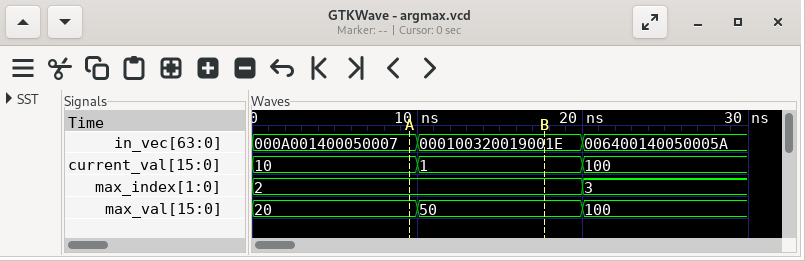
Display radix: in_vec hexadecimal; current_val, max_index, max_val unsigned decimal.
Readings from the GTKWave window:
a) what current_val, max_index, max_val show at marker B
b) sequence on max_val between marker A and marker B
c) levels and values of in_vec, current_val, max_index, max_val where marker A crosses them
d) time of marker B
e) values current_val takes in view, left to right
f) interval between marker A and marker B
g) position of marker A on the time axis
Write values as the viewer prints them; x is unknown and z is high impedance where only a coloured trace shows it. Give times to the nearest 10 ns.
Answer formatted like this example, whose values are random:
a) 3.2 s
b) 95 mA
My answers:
a) current_val=1, max_index=2, max_val=50
b) 20, 50
c) in_vec=000A001400050007, current_val=10, max_index=2, max_val=20
d) 20 ns
e) 10, 1, 100
f) 10 ns
g) 10 ns
